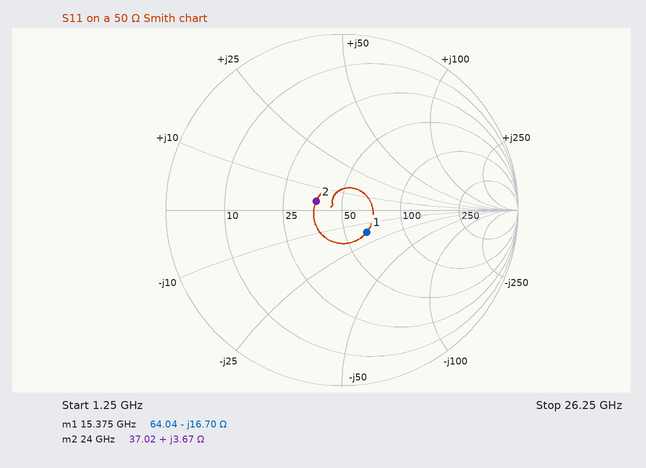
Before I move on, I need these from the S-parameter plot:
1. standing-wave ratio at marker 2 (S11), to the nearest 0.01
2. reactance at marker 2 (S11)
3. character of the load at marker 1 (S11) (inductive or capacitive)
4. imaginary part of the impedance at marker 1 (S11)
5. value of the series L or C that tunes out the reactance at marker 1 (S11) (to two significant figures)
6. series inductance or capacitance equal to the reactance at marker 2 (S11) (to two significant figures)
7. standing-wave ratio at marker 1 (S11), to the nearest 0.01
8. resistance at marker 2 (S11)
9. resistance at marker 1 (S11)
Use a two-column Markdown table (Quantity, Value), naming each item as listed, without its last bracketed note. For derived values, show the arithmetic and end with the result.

| Quantity | Value |
|---|---|
| standing-wave ratio at marker 2 (S11), to the nearest 0.01 | 1.37 |
| reactance at marker 2 | +3.67 Ω |
| character of the load at marker 1 (S11) | capacitive |
| imaginary part of the impedance at marker 1 | -16.70 Ω |
| value of the series L or C that tunes out the reactance at marker 1 (S11) | L = 16.7 Ω/(2π × 15.375 GHz) ≈ 173 pH, so 170 pH to two significant figures |
| series inductance or capacitance equal to the reactance at marker 2 (S11) | L = 3.67 Ω/(2π × 24 GHz) ≈ 24 pH |
| standing-wave ratio at marker 1 (S11), to the nearest 0.01 | 1.47 |
| resistance at marker 2 | 37.02 Ω |
| resistance at marker 1 | 64.04 Ω |
